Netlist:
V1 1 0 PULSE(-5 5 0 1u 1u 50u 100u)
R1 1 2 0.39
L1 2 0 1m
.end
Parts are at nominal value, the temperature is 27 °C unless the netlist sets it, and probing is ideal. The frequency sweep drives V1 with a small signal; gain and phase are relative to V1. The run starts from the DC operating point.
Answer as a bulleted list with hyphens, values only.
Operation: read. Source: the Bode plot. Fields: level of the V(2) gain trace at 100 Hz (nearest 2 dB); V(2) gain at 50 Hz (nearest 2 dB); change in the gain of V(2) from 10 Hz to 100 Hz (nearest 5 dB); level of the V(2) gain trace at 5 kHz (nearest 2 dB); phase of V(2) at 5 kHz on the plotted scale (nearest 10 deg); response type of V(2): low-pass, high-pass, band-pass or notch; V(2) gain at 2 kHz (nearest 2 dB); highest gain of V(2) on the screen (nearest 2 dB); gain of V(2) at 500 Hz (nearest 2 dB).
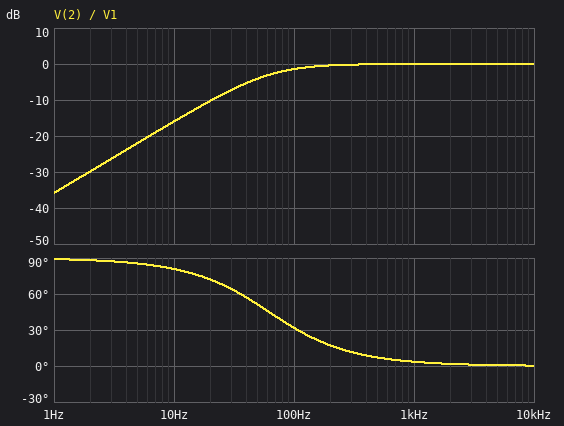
- -2 dB
- -4 dB
- 15 dB
- 0 dB
- 0 deg
- high-pass
- 0 dB
- 0 dB
- 0 dB
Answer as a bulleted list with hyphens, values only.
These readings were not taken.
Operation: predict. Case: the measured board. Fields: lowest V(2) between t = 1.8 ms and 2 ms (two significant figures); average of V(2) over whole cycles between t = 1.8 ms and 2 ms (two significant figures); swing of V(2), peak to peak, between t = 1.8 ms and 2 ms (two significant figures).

- -2.8 V
- 2.4 V
- 10 V
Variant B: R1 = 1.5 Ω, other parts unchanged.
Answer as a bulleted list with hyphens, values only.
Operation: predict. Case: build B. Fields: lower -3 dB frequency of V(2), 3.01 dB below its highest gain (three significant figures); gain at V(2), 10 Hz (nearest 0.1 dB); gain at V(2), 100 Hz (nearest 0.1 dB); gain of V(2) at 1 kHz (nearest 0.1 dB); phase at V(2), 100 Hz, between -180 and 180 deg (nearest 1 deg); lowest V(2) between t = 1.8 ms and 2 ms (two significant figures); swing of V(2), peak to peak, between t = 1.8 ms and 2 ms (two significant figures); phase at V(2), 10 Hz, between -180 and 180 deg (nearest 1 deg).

- 239 Hz
- -27.6 dB
- -8.3 dB
- -0.2 dB
- 67 deg
- -5.0 V
- 10 V
- 88 deg
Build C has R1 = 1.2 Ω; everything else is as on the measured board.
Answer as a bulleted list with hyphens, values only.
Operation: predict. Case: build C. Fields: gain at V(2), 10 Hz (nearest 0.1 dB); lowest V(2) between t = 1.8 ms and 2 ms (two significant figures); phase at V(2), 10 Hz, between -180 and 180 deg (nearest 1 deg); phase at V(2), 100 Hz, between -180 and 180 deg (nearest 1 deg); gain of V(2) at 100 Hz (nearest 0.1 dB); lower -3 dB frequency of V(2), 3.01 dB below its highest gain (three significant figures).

- -25.6 dB
- -4.8 V
- 87 deg
- 62 deg
- -6.7 dB
- 191 Hz
